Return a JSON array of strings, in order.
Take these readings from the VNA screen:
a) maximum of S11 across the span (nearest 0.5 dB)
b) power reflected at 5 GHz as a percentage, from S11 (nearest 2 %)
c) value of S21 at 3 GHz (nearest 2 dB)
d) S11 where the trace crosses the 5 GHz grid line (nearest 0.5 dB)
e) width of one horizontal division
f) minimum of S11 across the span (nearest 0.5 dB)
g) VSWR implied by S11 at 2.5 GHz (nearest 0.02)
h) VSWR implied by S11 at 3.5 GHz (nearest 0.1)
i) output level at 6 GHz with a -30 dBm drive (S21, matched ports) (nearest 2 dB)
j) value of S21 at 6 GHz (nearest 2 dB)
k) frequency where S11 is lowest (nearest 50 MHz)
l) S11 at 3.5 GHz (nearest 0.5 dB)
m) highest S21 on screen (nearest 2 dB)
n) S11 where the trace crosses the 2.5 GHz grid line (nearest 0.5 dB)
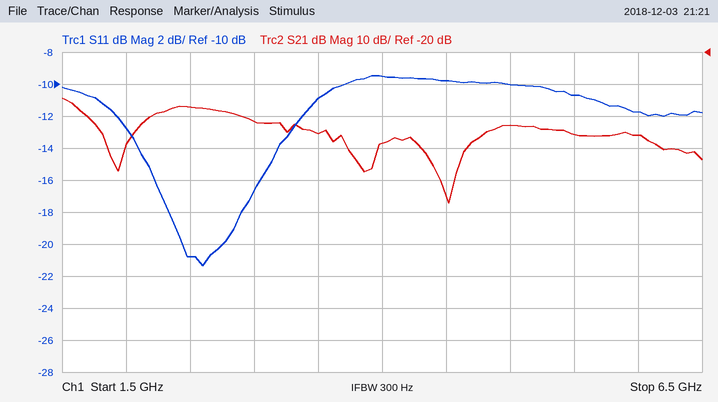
["-9.5 dB", "10 %", "-42 dB", "-10.0 dB", "500 MHz", "-21.5 dB", "1.20", "1.8", "-76 dBm", "-46 dB", "2.60 GHz", "-11.0 dB", "-34 dB", "-21.0 dB"]
